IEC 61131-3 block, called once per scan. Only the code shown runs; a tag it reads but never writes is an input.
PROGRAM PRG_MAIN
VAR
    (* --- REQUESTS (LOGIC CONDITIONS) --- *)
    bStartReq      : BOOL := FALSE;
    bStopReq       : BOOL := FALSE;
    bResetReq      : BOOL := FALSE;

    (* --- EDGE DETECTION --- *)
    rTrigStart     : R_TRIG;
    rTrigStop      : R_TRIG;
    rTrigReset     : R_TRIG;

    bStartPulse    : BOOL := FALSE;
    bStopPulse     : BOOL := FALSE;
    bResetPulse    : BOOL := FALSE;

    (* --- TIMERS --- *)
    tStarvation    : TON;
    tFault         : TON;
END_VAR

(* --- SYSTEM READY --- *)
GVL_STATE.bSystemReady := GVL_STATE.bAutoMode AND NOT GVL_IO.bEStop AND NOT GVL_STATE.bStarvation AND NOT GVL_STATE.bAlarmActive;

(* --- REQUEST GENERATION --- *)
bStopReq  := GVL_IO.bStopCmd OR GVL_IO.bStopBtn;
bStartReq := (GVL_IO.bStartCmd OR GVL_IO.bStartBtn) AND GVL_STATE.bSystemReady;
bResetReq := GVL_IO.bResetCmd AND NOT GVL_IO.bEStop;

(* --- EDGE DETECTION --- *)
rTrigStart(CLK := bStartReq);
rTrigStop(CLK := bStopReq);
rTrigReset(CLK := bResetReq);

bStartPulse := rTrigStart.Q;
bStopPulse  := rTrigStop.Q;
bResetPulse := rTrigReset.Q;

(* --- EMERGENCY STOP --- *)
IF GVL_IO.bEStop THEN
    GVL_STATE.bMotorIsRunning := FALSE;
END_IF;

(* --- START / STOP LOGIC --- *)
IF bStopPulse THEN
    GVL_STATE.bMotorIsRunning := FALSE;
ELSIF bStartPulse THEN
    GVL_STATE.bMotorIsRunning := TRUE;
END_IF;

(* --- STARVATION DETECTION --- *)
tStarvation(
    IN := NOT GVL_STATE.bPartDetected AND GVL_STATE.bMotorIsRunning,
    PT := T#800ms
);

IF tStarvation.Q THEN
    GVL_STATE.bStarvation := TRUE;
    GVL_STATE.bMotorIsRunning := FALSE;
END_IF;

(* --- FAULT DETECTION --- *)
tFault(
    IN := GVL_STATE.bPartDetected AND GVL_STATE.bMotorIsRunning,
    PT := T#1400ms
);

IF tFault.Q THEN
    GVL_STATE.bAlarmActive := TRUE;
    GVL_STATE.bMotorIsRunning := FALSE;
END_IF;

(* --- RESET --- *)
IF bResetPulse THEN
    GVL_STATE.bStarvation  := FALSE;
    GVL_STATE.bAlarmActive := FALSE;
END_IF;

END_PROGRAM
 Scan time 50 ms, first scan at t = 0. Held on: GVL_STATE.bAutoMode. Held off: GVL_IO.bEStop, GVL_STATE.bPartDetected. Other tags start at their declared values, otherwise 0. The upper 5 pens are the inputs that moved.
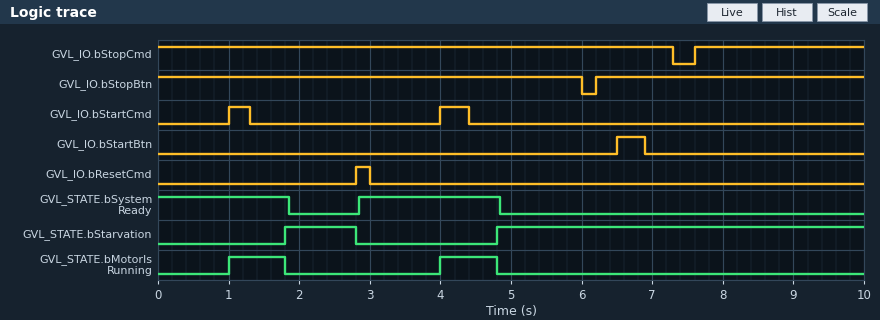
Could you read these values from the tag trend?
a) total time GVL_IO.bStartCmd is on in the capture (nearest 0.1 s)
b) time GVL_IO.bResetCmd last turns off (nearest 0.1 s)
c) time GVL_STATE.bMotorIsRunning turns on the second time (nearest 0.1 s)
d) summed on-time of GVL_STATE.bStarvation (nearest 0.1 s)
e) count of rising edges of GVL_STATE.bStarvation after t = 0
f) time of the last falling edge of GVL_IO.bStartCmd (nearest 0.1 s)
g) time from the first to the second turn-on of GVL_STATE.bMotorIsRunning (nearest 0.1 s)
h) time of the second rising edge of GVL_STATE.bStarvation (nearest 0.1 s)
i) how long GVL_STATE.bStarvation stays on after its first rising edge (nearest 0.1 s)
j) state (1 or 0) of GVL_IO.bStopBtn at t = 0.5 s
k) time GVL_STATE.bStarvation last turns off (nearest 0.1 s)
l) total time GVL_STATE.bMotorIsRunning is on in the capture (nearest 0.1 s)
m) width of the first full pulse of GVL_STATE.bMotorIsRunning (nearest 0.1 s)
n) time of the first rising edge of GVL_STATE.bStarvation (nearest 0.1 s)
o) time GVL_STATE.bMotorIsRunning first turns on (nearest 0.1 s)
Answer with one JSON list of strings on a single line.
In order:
["0.7 s", "3.0 s", "4.0 s", "6.2 s", "2", "4.4 s", "3.0 s", "4.8 s", "1.0 s", "1", "2.8 s", "1.6 s", "0.8 s", "1.8 s", "1.0 s"]
